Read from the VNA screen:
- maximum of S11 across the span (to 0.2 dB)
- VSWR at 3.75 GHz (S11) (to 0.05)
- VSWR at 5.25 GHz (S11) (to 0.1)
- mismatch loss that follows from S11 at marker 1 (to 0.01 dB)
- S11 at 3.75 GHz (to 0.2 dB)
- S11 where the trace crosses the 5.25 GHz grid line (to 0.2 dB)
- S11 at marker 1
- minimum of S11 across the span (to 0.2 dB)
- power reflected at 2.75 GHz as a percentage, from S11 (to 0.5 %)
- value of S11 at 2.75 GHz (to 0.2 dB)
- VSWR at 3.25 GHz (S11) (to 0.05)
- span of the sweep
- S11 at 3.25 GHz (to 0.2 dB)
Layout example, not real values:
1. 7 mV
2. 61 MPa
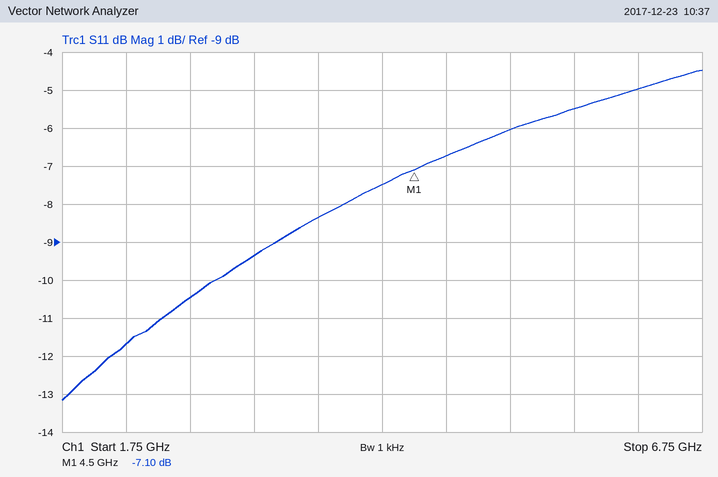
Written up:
1. -4.4 dB
2. 2.25
3. 3.0
4. 0.94 dB
5. -8.4 dB
6. -6.0 dB
7. -7.10 dB
8. -13.2 dB
9. 9.0 %
10. -10.4 dB
11. 2.05
12. 5 GHz
13. -9.4 dB
